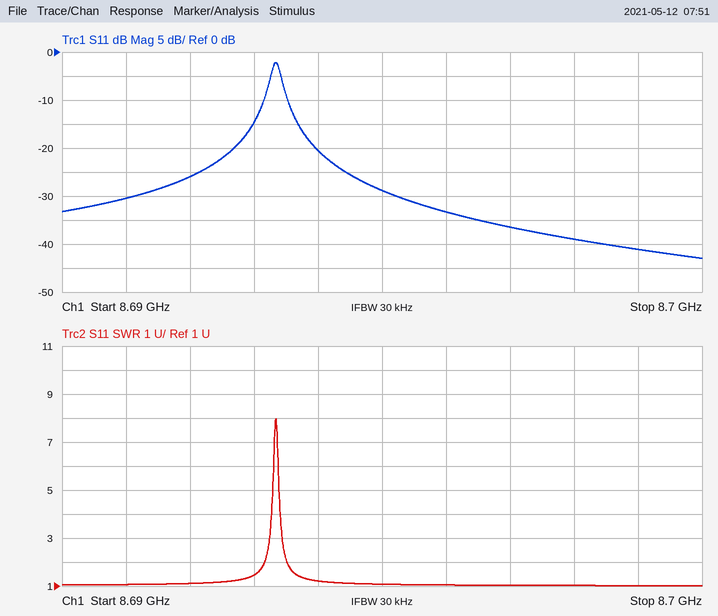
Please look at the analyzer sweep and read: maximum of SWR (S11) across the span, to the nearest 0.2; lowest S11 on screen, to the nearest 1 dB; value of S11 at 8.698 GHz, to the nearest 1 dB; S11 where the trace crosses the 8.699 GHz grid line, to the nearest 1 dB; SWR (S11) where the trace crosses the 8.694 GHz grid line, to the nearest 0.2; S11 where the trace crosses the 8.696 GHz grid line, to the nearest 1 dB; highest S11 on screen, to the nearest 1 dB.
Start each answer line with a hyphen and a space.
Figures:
- 8.0
- -43 dB
- -39 dB
- -41 dB
- 1.2
- -33 dB
- -2 dB
